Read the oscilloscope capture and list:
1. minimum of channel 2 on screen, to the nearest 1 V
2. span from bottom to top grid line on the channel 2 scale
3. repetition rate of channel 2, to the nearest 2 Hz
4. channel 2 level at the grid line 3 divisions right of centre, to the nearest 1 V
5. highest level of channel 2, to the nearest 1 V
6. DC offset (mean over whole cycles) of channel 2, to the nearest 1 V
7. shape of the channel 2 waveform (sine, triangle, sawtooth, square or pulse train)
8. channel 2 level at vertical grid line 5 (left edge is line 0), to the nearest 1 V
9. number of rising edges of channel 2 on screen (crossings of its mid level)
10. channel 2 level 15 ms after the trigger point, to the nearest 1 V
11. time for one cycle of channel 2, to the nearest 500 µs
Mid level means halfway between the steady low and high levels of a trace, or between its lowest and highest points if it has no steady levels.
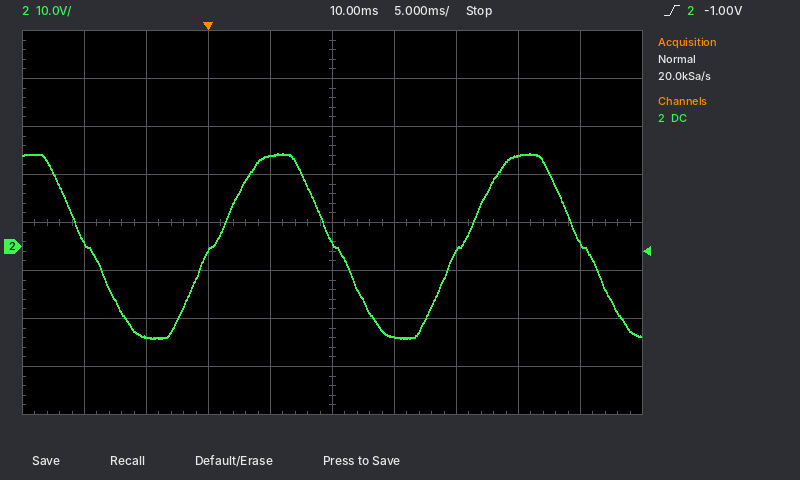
-19 V
80 V
50 Hz
19 V
19 V
0 V
sine
1 V
2
-19 V
20.0 ms
